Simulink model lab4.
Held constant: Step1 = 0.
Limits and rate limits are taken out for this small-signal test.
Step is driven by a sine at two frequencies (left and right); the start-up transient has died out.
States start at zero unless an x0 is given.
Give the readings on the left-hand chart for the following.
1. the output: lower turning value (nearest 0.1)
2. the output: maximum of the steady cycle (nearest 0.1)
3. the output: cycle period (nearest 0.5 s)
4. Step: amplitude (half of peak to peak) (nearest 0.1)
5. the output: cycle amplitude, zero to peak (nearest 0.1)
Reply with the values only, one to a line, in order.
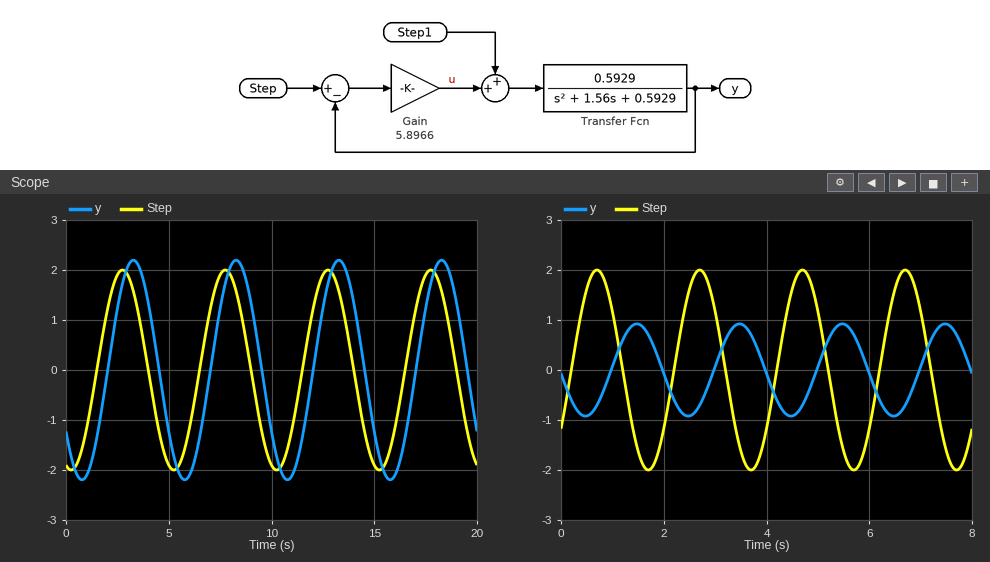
-2.2
2.2
5.0 s
2.0
2.2
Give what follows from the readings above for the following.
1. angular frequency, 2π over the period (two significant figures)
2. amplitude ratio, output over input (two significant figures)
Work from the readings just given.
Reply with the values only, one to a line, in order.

1.3 rad/s
1.1
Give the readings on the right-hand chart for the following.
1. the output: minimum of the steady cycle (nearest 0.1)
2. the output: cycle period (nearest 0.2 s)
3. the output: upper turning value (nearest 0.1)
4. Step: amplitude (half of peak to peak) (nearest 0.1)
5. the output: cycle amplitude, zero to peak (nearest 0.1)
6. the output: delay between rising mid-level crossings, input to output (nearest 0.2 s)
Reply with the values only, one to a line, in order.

-0.9
2.0 s
0.9
2.0
0.9
0.8 s
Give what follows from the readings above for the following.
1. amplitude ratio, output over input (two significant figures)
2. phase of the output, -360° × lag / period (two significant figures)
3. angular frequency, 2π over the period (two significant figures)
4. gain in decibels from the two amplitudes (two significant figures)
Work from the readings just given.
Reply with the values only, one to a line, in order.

0.45
-140°
3.1 rad/s
-6.9 dB
